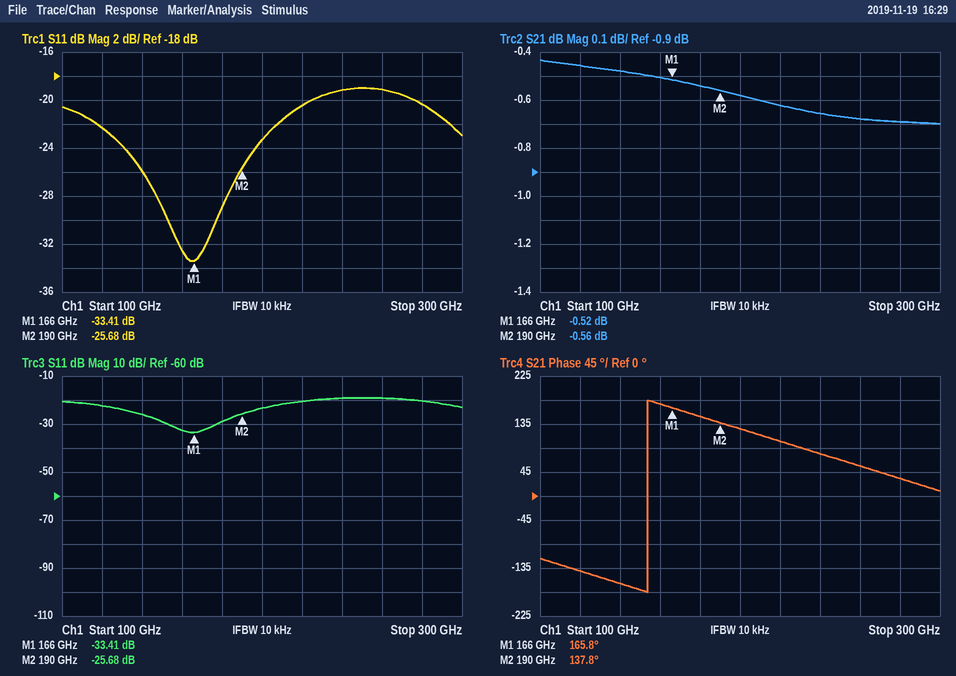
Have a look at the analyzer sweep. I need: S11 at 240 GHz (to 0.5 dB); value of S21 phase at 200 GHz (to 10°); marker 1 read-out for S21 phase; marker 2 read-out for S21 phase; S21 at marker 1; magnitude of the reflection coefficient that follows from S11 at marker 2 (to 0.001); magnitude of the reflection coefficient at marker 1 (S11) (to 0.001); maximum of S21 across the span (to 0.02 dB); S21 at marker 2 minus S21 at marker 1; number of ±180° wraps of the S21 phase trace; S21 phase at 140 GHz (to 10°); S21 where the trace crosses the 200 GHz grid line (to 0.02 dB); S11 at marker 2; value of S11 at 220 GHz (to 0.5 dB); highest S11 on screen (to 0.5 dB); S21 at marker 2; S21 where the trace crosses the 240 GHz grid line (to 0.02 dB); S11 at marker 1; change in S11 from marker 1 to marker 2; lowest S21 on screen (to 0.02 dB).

-19.0 dB
130°
165.8°
137.8°
-0.52 dB
0.052
0.021
-0.44 dB
-0.04 dB
1
-160°
-0.58 dB
-25.68 dB
-20.5 dB
-19.0 dB
-0.56 dB
-0.66 dB
-33.41 dB
7.73 dB
-0.70 dB
